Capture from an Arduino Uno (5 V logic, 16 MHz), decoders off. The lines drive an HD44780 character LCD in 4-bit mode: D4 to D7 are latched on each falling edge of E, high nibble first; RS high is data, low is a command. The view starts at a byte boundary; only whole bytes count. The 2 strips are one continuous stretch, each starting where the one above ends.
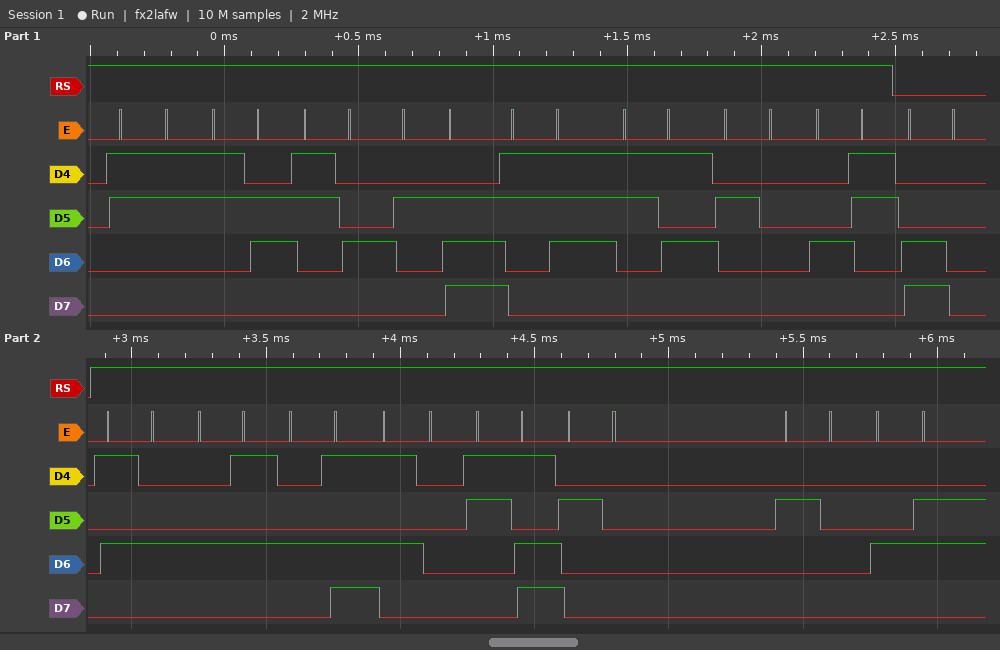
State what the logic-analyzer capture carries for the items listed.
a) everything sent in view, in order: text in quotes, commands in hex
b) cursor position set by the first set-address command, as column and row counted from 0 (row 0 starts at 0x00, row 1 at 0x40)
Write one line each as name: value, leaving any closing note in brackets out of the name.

everything sent in view, in order: text in quotes, commands in hex: "364.75 C" 0xC0 "TEMP=  F"
cursor position set by the first set-address command, as column and row counted from 0: column 0, row 1
